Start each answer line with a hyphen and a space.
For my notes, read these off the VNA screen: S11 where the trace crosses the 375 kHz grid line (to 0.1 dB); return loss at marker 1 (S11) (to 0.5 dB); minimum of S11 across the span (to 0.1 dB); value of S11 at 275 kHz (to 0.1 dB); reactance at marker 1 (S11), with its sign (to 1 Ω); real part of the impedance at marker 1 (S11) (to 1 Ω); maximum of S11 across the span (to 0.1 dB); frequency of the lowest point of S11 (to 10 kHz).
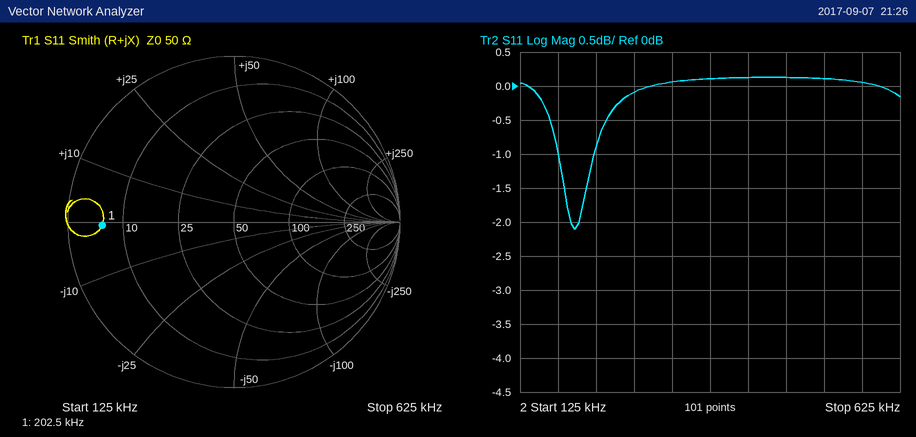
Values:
- 0.1 dB
- 2.0 dB
- -2.1 dB
- -0.1 dB
- -1 Ω
- 6 Ω
- 0.1 dB
- 200 kHz
